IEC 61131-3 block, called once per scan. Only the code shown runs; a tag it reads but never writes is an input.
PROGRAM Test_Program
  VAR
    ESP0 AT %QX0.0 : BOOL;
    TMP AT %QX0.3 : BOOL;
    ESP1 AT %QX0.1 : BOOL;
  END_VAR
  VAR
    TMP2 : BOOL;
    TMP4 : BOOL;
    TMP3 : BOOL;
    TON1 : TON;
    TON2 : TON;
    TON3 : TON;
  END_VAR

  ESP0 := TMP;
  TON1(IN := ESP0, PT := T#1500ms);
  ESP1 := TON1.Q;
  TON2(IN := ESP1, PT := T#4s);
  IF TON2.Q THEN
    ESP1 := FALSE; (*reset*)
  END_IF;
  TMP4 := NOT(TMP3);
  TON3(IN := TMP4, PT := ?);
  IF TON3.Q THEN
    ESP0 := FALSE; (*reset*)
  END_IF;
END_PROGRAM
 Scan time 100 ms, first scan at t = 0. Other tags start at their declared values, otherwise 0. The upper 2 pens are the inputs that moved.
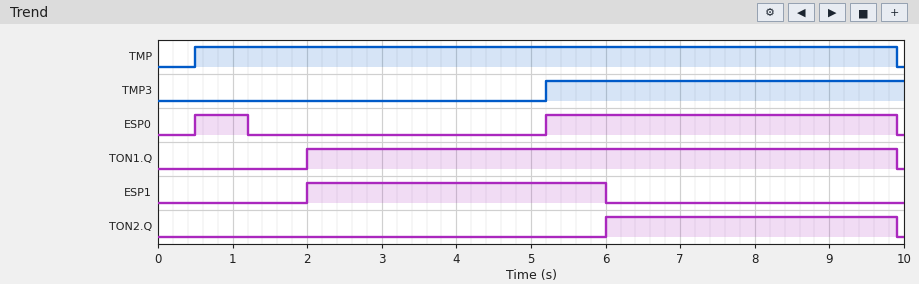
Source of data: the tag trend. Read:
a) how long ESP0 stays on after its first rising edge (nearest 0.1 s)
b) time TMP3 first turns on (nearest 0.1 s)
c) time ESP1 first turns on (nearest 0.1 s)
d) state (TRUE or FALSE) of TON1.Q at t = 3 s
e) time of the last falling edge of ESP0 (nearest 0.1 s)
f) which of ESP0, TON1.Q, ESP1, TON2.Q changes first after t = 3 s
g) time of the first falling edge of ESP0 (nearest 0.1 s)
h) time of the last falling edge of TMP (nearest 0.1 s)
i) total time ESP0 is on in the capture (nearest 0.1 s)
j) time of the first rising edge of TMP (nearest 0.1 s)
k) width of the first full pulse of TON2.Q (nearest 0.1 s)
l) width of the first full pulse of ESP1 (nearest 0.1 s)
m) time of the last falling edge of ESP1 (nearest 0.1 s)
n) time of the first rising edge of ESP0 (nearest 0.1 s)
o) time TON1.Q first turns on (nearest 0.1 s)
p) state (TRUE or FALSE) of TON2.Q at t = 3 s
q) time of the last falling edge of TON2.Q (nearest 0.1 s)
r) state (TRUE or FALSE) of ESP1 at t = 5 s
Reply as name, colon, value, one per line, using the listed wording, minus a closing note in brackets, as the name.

how long ESP0 stays on after its first rising edge: 0.7 s
time TMP3 first turns on: 5.2 s
time ESP1 first turns on: 2.0 s
state (TRUE or FALSE) of TON1.Q at t = 3 s: TRUE
time of the last falling edge of ESP0: 9.9 s
which of ESP0, TON1.Q, ESP1, TON2.Q changes first after t = 3 s: ESP0
time of the first falling edge of ESP0: 1.2 s
time of the last falling edge of TMP: 9.9 s
total time ESP0 is on in the capture: 5.4 s
time of the first rising edge of TMP: 0.5 s
width of the first full pulse of TON2.Q: 3.9 s
width of the first full pulse of ESP1: 4.0 s
time of the last falling edge of ESP1: 6.0 s
time of the first rising edge of ESP0: 0.5 s
time TON1.Q first turns on: 2.0 s
state (TRUE or FALSE) of TON2.Q at t = 3 s: FALSE
time of the last falling edge of TON2.Q: 9.9 s
state (TRUE or FALSE) of ESP1 at t = 5 s: TRUE
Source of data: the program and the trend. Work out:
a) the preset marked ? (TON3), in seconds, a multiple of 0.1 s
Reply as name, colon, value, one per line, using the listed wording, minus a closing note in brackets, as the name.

the preset marked ? (TON3), in seconds, a multiple of 0.1 s: 1.2 s
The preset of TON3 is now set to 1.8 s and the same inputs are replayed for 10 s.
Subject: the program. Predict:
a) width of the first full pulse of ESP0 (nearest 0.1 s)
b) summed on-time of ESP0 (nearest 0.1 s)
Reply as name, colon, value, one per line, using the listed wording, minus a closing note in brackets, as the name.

width of the first full pulse of ESP0: 1.3 s
summed on-time of ESP0: 6.0 s
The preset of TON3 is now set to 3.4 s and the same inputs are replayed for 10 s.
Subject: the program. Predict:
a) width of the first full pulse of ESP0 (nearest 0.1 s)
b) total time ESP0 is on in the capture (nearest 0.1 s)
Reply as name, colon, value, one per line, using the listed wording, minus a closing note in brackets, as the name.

width of the first full pulse of ESP0: 2.9 s
total time ESP0 is on in the capture: 7.6 s
